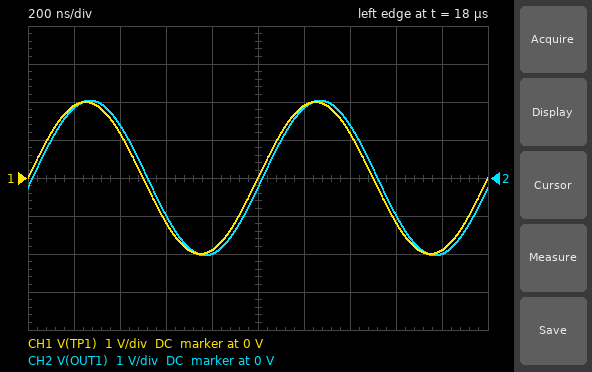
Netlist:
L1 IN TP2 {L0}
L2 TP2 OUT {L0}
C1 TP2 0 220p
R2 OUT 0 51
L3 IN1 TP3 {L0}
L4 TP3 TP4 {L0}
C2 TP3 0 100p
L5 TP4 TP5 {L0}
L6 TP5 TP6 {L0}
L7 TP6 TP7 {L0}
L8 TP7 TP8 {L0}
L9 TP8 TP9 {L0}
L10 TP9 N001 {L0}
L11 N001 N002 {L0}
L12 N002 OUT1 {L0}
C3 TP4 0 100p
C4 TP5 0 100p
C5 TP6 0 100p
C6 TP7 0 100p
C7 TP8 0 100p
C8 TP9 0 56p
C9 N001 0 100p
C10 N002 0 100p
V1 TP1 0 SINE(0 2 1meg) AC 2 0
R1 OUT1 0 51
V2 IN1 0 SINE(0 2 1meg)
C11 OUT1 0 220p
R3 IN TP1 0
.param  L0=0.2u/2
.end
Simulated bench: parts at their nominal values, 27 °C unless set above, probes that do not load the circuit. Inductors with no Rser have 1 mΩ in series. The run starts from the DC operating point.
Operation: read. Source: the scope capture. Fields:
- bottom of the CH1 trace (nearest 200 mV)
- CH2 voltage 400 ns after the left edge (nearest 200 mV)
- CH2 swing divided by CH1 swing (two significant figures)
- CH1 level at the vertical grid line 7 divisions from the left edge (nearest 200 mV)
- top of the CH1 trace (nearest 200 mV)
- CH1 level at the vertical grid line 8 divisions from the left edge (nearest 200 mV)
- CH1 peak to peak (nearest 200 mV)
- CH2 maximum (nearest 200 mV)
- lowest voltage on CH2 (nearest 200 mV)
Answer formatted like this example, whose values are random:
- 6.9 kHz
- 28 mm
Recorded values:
- -2.0 V
- 1.4 V
- 1.0
- 1.2 V
- 2.0 V
- -1.2 V
- 4.0 V
- 2.0 V
- -2.0 V
